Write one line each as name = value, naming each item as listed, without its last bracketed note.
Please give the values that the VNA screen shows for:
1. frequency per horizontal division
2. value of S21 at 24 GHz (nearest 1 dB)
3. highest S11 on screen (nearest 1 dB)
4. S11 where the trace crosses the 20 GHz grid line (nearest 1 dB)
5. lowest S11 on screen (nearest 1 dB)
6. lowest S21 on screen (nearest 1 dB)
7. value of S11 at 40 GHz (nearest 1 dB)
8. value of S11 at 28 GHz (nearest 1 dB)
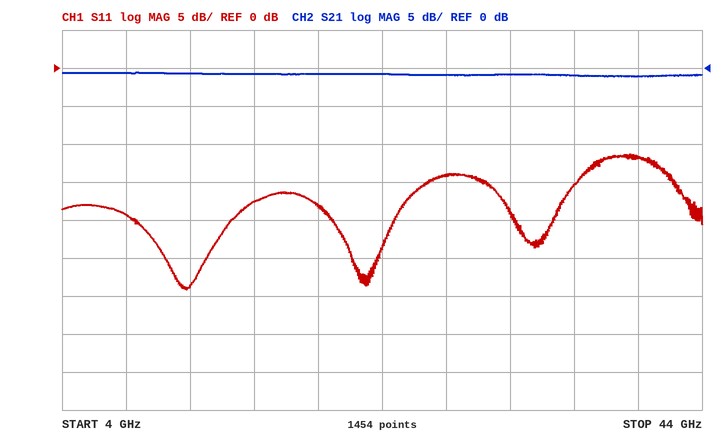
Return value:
frequency per horizontal division = 4 GHz
value of S21 at 24 GHz = -1 dB
highest S11 on screen = -11 dB
S11 where the trace crosses the 20 GHz grid line = -18 dB
lowest S11 on screen = -29 dB
lowest S21 on screen = -1 dB
value of S11 at 40 GHz = -12 dB
value of S11 at 28 GHz = -14 dB
